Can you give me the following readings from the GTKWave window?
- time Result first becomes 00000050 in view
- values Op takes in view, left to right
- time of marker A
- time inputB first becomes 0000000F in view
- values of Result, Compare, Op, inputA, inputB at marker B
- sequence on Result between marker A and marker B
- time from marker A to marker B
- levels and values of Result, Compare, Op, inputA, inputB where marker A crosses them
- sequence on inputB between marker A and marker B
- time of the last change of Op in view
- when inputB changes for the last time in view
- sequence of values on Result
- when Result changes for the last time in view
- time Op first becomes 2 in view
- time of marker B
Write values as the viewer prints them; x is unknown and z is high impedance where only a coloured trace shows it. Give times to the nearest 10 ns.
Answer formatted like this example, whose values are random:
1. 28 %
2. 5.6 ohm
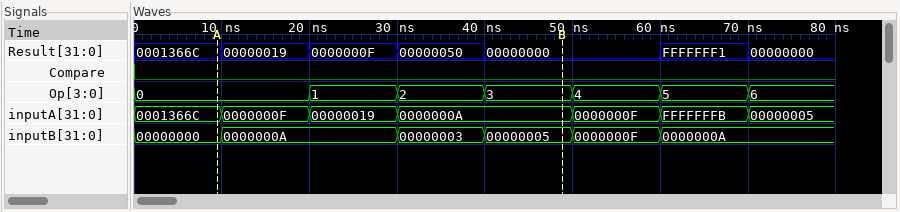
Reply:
1. 30 ns
2. 0, 1, 2, 3, 4, 5, 6
3. 10 ns
4. 50 ns
5. Result=00000000, Compare=0, Op=3, inputA=0000000A, inputB=00000005
6. 0001366C, 00000019, 0000000F, 00000050, 00000000
7. 40 ns
8. Result=0001366C, Compare=0, Op=0, inputA=0001366C, inputB=00000000
9. 00000000, 0000000A, 00000003, 00000005
10. 70 ns
11. 60 ns
12. 0001366C, 00000019, 0000000F, 00000050, 00000000, FFFFFFF1, 00000000
13. 70 ns
14. 30 ns
15. 50 ns
